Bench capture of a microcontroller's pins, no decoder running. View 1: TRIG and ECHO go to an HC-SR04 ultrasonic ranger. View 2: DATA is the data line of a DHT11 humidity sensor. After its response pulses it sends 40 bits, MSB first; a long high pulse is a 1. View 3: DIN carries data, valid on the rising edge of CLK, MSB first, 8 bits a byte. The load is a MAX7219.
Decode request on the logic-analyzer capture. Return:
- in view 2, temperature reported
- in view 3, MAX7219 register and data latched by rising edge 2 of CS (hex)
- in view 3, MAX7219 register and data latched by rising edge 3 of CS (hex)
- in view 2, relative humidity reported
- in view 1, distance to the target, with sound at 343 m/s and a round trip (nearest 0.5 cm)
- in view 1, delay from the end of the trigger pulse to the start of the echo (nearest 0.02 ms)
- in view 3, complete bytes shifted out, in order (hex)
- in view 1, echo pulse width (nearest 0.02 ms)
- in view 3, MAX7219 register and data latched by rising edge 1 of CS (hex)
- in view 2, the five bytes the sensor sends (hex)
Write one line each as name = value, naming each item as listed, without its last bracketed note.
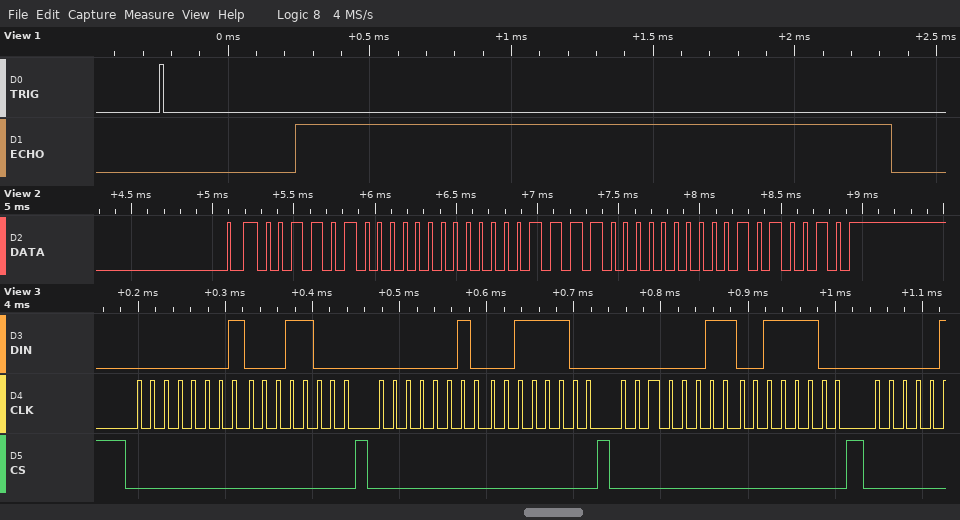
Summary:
in view 2, temperature reported = 30.0 °C
in view 3, MAX7219 register and data latched by rising edge 2 of CS = register 0x2, data 0x3C
in view 3, MAX7219 register and data latched by rising edge 3 of CS = register 0x3, data 0x3C
in view 2, relative humidity reported = 52 %
in view 1, distance to the target, with sound at 343 m/s and a round trip = 36 cm
in view 1, delay from the end of the trigger pulse to the start of the echo = 0.46 ms
in view 3, complete bytes shifted out, in order = 0x01 0x18 0x02 0x3C 0x03 0x3C
in view 1, echo pulse width = 2.10 ms
in view 3, MAX7219 register and data latched by rising edge 1 of CS = register 0x1, data 0x18
in view 2, the five bytes the sensor sends = 34 00 1E 00 52
